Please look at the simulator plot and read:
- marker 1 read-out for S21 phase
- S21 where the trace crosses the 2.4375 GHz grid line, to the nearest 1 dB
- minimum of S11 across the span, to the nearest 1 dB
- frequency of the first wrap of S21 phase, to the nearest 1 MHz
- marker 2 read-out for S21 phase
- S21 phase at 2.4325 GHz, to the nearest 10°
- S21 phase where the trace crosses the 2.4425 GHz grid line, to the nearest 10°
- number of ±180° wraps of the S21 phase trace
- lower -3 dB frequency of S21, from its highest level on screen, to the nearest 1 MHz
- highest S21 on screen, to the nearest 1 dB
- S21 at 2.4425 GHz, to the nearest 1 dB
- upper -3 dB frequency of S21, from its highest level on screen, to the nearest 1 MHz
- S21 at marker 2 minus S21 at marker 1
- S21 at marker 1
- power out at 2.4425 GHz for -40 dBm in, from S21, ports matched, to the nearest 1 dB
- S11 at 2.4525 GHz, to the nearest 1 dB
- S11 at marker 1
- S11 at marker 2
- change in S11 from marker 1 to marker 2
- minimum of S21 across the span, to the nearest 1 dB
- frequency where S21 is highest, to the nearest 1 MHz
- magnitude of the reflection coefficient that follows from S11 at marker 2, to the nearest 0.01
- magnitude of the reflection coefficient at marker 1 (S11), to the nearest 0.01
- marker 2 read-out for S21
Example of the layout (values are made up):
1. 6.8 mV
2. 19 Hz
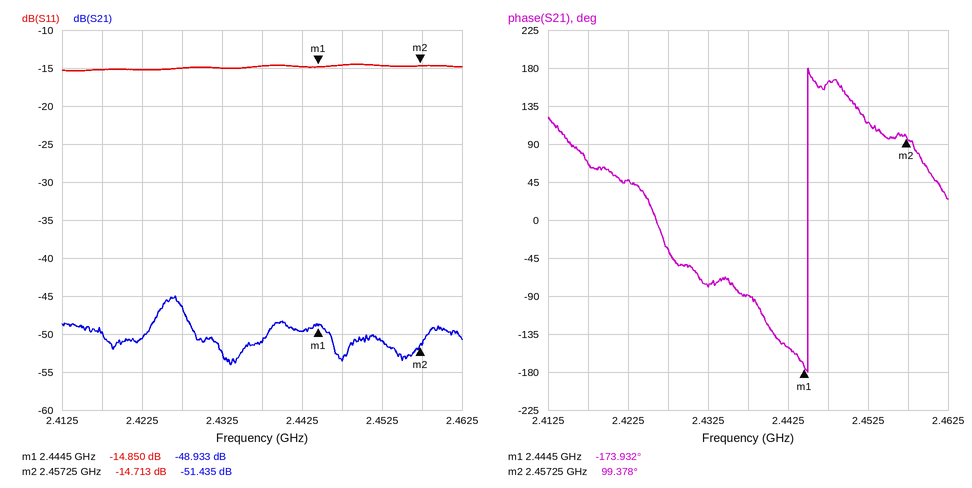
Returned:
1. -173.932°
2. -51 dB
3. -15 dB
4. 2.445 GHz
5. 99.378°
6. -80°
7. -150°
8. 1
9. 2.424 GHz
10. -45 dB
11. -50 dB
12. 2.428 GHz
13. -2.502 dB
14. -48.933 dB
15. -90 dBm
16. -15 dB
17. -14.850 dB
18. -14.713 dB
19. 0.137 dB
20. -54 dB
21. 2.427 GHz
22. 0.18
23. 0.18
24. -51.435 dB
